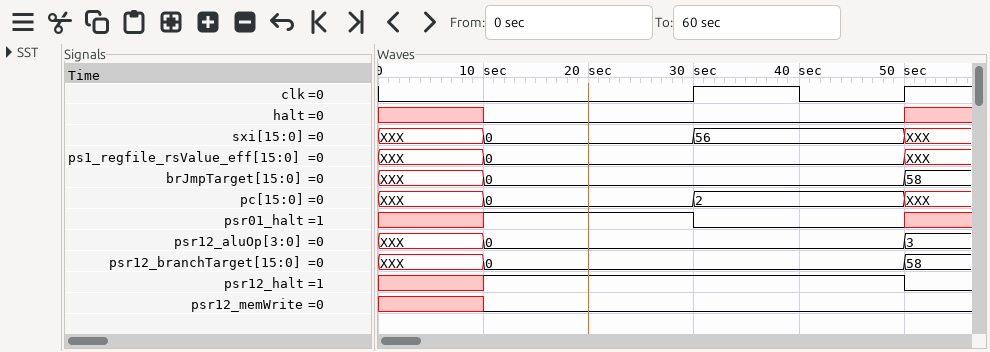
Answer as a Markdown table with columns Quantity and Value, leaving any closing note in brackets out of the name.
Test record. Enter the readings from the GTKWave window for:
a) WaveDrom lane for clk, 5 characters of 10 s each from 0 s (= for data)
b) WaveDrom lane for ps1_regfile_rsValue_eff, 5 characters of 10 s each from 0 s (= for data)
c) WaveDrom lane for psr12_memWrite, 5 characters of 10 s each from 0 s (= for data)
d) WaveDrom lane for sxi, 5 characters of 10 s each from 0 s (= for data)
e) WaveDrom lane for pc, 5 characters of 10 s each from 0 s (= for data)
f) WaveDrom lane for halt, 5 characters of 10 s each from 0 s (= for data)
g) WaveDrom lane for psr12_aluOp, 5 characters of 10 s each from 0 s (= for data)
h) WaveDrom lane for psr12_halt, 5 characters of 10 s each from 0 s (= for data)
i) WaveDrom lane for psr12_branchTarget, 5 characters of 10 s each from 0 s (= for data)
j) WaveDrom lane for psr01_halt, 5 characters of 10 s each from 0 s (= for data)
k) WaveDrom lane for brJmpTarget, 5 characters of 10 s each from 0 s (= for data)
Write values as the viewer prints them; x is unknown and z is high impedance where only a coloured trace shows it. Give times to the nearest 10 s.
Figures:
| Quantity | Value |
|---|---|
| WaveDrom lane for clk, 5 characters of 10 s each from 0 s | {name: 'clk', wave: '0..10'} |
| WaveDrom lane for ps1_regfile_rsValue_eff, 5 characters of 10 s each from 0 s | {name: 'ps1_regfile_rsValue_eff', wave: 'x=...', data: '0'} |
| WaveDrom lane for psr12_memWrite, 5 characters of 10 s each from 0 s | {name: 'psr12_memWrite', wave: 'x0...'} |
| WaveDrom lane for sxi, 5 characters of 10 s each from 0 s | {name: 'sxi', wave: 'x=.=.', data: '0 56'} |
| WaveDrom lane for pc, 5 characters of 10 s each from 0 s | {name: 'pc', wave: 'x=.=.', data: '0 2'} |
| WaveDrom lane for halt, 5 characters of 10 s each from 0 s | {name: 'halt', wave: 'x0...'} |
| WaveDrom lane for psr12_aluOp, 5 characters of 10 s each from 0 s | {name: 'psr12_aluOp', wave: 'x=...', data: '0'} |
| WaveDrom lane for psr12_halt, 5 characters of 10 s each from 0 s | {name: 'psr12_halt', wave: 'x1...'} |
| WaveDrom lane for psr12_branchTarget, 5 characters of 10 s each from 0 s | {name: 'psr12_branchTarget', wave: 'x=...', data: '0'} |
| WaveDrom lane for psr01_halt, 5 characters of 10 s each from 0 s | {name: 'psr01_halt', wave: 'x1.0.'} |
| WaveDrom lane for brJmpTarget, 5 characters of 10 s each from 0 s | {name: 'brJmpTarget', wave: 'x=...', data: '0'} |
